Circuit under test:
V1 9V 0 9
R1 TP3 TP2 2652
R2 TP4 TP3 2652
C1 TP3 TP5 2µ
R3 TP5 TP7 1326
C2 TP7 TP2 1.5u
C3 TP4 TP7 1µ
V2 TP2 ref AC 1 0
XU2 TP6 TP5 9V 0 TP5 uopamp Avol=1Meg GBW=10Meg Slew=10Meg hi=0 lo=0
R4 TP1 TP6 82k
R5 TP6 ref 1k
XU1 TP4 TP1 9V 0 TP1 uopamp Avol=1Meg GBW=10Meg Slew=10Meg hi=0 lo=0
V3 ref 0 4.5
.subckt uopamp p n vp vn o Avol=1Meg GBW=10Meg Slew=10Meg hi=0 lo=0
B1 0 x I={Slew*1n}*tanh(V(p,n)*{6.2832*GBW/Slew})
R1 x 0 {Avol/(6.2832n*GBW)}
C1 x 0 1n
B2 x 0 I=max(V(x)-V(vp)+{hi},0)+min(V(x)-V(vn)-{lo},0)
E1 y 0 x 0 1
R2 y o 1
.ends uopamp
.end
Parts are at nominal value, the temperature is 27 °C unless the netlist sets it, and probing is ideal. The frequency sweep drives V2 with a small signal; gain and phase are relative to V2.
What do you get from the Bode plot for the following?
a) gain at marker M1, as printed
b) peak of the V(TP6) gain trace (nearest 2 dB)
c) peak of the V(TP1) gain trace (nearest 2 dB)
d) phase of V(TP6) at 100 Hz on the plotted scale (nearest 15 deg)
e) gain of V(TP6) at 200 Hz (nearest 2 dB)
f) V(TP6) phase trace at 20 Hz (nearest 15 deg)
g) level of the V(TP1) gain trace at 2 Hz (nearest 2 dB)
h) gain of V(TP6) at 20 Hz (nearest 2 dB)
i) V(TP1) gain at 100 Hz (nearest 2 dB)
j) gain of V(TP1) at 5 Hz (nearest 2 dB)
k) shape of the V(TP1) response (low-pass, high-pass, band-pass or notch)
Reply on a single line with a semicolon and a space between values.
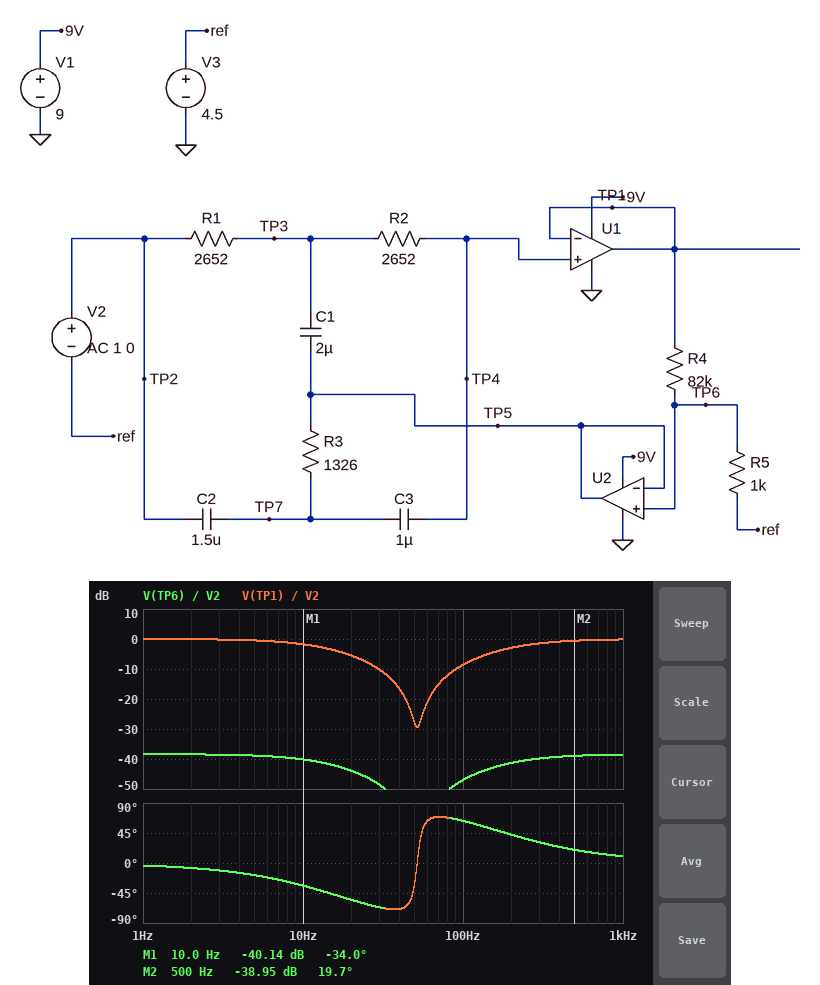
-40.14 dB; -38 dB; 0 dB; 60 deg; -42 dB; -60 deg; 0 dB; -44 dB; -8 dB; 0 dB; notch
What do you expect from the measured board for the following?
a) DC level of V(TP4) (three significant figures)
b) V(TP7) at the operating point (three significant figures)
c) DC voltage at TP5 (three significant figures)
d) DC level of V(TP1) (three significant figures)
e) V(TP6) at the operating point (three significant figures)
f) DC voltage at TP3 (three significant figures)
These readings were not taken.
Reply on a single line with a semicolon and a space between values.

4.50 V; 4.50 V; 4.50 V; 4.50 V; 4.50 V; 4.50 V
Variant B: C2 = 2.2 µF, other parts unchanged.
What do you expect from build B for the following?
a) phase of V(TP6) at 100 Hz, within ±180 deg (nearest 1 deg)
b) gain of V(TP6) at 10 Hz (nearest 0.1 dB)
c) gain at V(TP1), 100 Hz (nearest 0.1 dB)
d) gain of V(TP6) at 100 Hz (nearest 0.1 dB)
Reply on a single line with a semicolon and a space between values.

53 deg; -40.3 dB; -6.6 dB; -45.0 dB
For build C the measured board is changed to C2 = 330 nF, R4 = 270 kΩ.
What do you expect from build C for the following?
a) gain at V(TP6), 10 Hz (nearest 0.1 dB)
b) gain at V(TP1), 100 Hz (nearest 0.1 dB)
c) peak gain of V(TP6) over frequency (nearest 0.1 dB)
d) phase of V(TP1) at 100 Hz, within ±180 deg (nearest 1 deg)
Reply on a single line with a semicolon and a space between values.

-50.2 dB; -28.3 dB; -48.7 dB; 136 deg
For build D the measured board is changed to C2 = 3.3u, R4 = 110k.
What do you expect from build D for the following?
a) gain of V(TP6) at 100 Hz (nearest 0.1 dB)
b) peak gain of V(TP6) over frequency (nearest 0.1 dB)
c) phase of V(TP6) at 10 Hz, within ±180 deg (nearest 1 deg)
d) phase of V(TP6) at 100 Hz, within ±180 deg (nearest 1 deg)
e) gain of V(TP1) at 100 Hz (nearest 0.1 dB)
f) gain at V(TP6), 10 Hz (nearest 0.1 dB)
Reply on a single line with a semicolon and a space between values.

-46.1 dB; -40.9 dB; -33 deg; 44 deg; -5.2 dB; -43.1 dB
